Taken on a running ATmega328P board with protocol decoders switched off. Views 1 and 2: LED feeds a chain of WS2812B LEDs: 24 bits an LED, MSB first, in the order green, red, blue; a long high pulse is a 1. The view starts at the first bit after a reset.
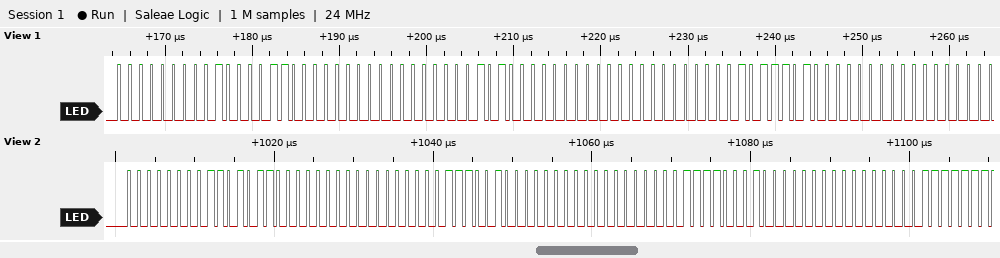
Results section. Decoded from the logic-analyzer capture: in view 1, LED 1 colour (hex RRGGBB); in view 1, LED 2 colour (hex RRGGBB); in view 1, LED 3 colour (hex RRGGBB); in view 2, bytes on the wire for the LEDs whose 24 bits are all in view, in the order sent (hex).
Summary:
#430000
#500000
#5D0000
00 D6 00 00 E4 00 00 F1 00
